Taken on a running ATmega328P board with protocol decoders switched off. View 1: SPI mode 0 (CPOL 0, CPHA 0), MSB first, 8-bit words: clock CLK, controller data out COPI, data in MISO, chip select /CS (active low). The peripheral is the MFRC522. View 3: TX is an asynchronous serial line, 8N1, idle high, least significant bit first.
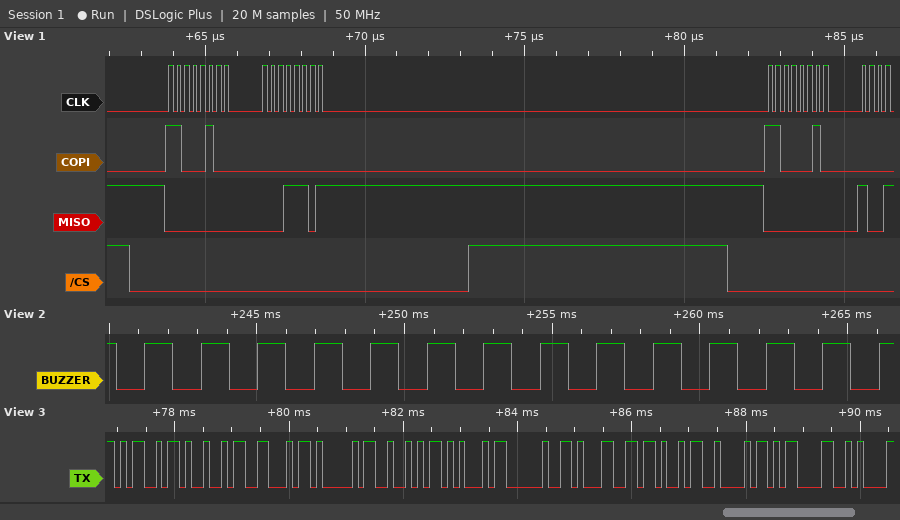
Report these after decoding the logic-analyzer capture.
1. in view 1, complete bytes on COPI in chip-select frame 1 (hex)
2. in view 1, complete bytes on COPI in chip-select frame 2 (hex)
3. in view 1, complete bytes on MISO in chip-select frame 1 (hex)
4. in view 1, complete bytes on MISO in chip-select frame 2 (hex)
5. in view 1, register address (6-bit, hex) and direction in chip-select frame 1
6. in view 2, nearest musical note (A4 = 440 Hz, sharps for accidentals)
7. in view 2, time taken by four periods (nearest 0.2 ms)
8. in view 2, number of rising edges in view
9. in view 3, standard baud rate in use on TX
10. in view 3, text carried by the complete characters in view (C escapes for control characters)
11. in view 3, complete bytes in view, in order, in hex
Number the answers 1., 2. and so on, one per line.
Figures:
1. C4 00
2. C2
3. 00 1D
4. 00
5. 0x22 read
6. C5
7. 7.6 ms
8. 14
9. 9600 baud
10. "MIFARE 1KB\r\n"
11. 4D 49 46 41 52 45 20 31 4B 42 0D 0A
